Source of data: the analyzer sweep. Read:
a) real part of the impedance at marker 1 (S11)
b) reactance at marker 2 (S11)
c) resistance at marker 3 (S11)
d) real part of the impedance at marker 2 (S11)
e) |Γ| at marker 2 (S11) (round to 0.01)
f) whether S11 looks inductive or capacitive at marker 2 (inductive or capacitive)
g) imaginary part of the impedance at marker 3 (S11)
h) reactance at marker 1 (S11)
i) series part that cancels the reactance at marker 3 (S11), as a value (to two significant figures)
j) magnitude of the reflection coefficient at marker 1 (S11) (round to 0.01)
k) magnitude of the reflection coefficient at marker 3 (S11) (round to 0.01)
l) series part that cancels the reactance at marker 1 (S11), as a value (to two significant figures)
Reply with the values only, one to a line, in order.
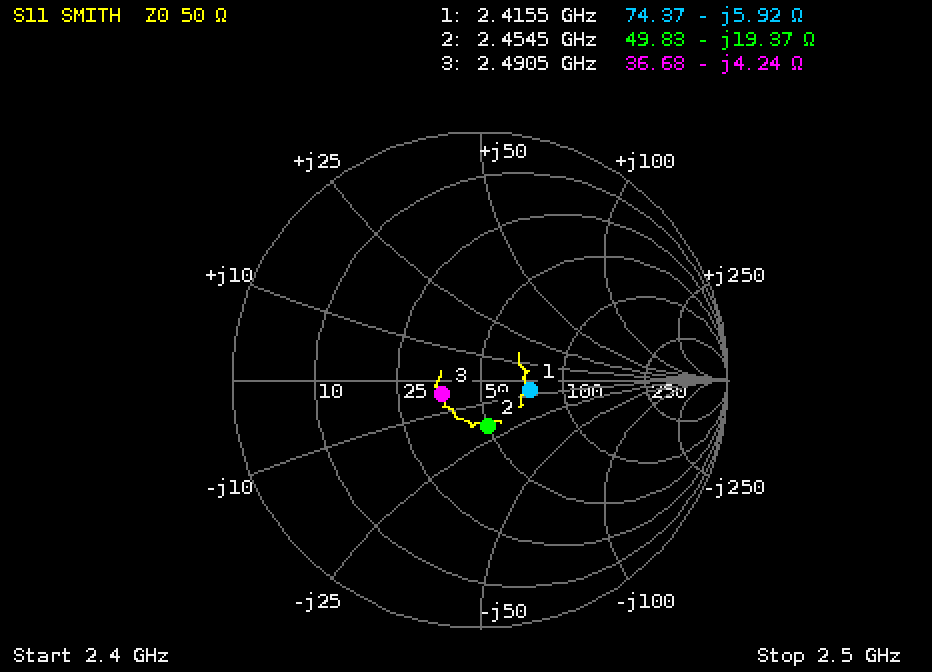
74.37 Ω
-19.37 Ω
36.68 Ω
49.83 Ω
0.19
capacitive
-4.24 Ω
-5.92 Ω
270 pH
0.20
0.16
390 pH
